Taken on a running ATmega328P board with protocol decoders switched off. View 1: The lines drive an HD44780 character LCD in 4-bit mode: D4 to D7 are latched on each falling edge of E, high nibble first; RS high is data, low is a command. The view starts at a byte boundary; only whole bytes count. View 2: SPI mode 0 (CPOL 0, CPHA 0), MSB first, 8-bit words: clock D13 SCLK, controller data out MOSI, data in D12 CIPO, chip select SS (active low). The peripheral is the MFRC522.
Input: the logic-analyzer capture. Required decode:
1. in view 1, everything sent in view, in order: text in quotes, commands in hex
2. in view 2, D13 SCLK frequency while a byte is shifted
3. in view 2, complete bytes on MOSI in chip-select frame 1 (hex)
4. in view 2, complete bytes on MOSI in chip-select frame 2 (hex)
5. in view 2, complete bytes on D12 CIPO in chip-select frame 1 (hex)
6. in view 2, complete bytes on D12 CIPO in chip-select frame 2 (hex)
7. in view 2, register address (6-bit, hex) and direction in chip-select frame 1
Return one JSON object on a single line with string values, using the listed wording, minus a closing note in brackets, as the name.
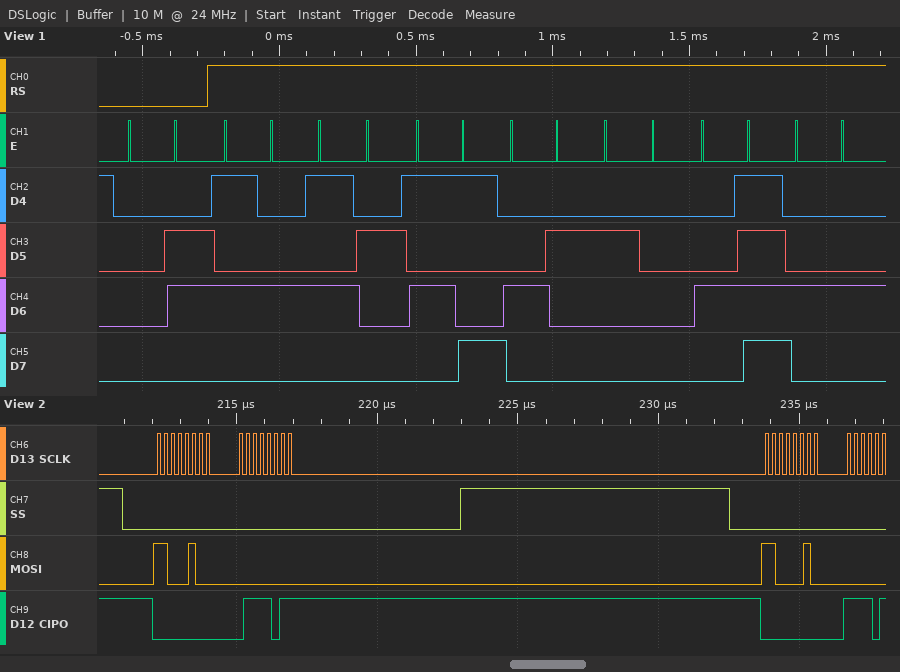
{"in view 1, everything sent in view, in order: text in quotes, commands in hex": "0x06 \"TRYB OD\"", "in view 2, D13 SCLK frequency while a byte is shifted": "4 MHz", "in view 2, complete bytes on MOSI in chip-select frame 1": "C4 00", "in view 2, complete bytes on MOSI in chip-select frame 2": "C2", "in view 2, complete bytes on D12 CIPO in chip-select frame 1": "00 7B", "in view 2, complete bytes on D12 CIPO in chip-select frame 2": "00", "in view 2, register address (6-bit, hex) and direction in chip-select frame 1": "0x22 read"}
